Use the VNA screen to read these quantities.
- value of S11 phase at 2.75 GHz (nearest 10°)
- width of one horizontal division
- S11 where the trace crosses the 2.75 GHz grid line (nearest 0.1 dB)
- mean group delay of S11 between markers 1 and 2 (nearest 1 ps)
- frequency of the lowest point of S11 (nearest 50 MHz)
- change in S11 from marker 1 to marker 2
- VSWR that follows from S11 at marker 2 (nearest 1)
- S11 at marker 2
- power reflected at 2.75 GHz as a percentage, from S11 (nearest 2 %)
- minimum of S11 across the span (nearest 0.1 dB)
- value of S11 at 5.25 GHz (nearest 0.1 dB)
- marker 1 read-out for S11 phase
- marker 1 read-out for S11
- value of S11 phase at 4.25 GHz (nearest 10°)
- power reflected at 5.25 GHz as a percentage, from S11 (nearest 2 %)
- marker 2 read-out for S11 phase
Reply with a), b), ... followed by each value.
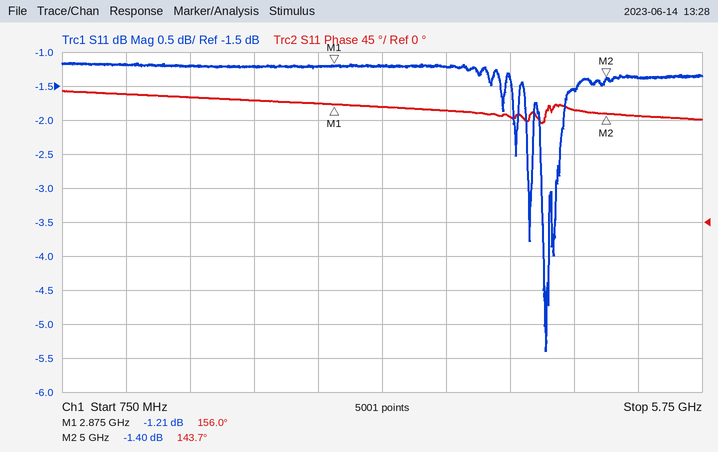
a) 160°
b) 500 MHz
c) -1.2 dB
d) 16 ps
e) 4.55 GHz
f) -0.19 dB
g) 12
h) -1.40 dB
i) 76 %
j) -5.4 dB
k) -1.4 dB
l) 156.0°
m) -1.21 dB
n) 140°
o) 72 %
p) 143.7°
